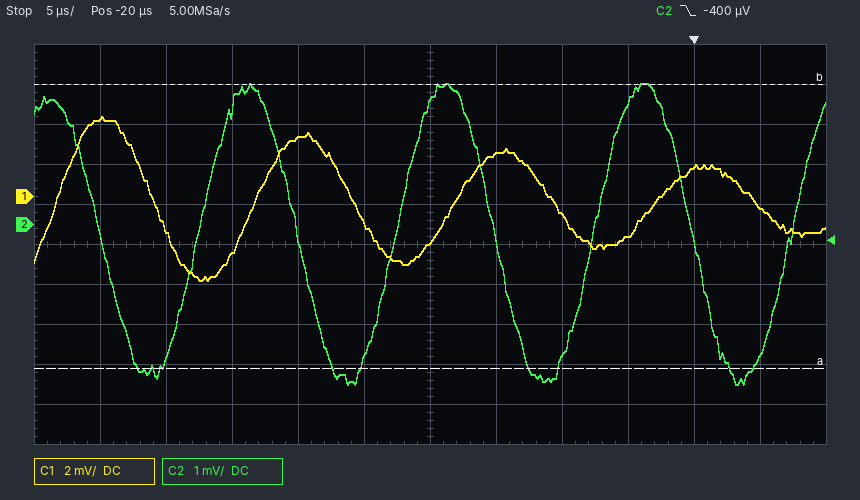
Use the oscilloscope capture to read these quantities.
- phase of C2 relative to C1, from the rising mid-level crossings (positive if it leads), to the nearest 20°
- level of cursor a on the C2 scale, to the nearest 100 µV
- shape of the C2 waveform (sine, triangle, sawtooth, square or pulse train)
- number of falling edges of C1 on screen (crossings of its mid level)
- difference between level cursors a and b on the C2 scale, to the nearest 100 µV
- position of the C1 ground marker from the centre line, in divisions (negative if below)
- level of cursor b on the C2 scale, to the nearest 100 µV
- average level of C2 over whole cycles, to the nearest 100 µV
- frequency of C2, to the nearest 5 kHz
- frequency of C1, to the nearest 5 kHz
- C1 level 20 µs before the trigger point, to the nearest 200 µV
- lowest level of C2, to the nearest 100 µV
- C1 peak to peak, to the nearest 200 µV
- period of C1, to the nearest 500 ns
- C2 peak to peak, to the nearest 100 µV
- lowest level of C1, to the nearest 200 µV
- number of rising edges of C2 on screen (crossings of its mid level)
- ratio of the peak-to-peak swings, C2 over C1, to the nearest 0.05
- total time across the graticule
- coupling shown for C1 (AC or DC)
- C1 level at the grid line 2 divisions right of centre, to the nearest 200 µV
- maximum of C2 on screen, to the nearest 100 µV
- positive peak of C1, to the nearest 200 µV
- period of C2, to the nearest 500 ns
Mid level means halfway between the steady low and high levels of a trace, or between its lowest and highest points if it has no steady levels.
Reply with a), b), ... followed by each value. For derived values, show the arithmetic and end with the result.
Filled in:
a) +120°
b) -3.6 mV
c) sine
d) 4
e) 7.1 mV
f) +1.2 div
g) 3.5 mV
h) (3.5 mV + (-4.0 mV)) / 2 ≈ -250 µV, so -200 µV to the nearest 100 µV
i) 1 / 15.0 µs ≈ 66.7 kHz, so 65 kHz to the nearest 5 kHz
j) 1 / 15.0 µs ≈ 66.7 kHz, so 65 kHz to the nearest 5 kHz
k) -2.2 mV
l) -4.0 mV
m) 4.0 mV − (-4.2 mV) = 8.2 mV
n) 15.0 µs
o) 3.5 mV − (-4.0 mV) = 7.5 mV
p) -4.2 mV
q) 4
r) 7.5 mV / 8.2 mV ≈ 0.915, so 0.90 to the nearest 0.05
s) 60 µs
t) DC
u) -1.0 mV
v) 3.5 mV
w) 4.0 mV
x) 15.0 µs
